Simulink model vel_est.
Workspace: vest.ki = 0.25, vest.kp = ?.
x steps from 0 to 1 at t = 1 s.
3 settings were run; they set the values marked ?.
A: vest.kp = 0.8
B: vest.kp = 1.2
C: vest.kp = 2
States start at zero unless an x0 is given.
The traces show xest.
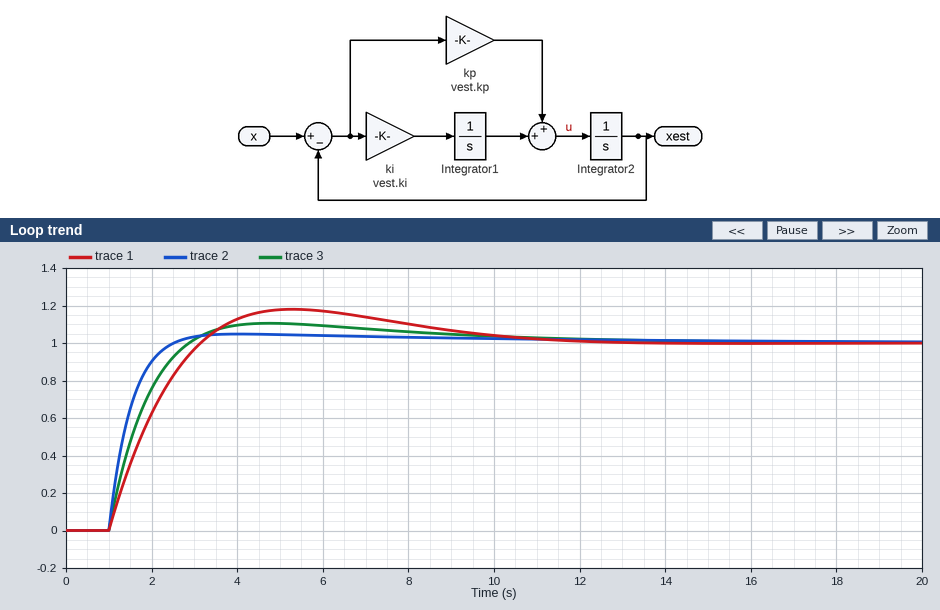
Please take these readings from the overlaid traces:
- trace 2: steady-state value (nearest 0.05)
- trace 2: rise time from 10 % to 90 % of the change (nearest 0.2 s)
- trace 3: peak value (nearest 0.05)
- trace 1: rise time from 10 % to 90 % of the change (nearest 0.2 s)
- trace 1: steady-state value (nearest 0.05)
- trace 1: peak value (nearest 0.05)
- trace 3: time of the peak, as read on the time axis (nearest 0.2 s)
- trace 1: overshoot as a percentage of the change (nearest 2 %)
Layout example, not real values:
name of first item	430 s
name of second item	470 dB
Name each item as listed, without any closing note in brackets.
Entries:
trace 2: steady-state value	1.00
trace 2: rise time from 10 % to 90 % of the change	1.0 s
trace 3: peak value	1.10
trace 1: rise time from 10 % to 90 % of the change	1.6 s
trace 1: steady-state value	1.00
trace 1: peak value	1.20
trace 3: time of the peak, as read on the time axis	4.8 s
trace 1: overshoot as a percentage of the change	18 %
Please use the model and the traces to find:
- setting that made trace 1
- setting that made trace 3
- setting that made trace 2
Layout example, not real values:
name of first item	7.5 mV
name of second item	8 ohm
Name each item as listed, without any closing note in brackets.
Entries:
setting that made trace 1	A
setting that made trace 3	B
setting that made trace 2	C
